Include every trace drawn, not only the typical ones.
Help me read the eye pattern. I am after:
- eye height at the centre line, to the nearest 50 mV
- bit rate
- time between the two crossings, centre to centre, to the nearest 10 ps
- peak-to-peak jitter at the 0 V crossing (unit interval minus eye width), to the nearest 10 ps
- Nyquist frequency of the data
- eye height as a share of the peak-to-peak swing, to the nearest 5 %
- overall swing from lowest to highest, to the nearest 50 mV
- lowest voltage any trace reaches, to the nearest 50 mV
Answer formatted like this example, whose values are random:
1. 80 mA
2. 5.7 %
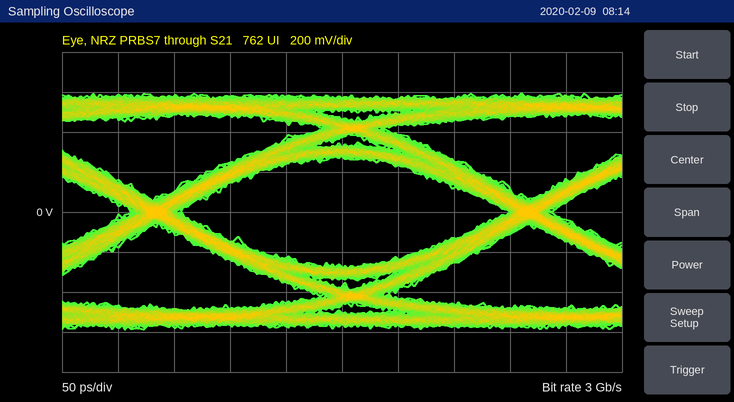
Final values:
1. 550 mV
2. 3 Gb/s
3. 330 ps
4. 40 ps
5. 1.5 GHz
6. 45 %
7. 1.20 V
8. -600 mV
